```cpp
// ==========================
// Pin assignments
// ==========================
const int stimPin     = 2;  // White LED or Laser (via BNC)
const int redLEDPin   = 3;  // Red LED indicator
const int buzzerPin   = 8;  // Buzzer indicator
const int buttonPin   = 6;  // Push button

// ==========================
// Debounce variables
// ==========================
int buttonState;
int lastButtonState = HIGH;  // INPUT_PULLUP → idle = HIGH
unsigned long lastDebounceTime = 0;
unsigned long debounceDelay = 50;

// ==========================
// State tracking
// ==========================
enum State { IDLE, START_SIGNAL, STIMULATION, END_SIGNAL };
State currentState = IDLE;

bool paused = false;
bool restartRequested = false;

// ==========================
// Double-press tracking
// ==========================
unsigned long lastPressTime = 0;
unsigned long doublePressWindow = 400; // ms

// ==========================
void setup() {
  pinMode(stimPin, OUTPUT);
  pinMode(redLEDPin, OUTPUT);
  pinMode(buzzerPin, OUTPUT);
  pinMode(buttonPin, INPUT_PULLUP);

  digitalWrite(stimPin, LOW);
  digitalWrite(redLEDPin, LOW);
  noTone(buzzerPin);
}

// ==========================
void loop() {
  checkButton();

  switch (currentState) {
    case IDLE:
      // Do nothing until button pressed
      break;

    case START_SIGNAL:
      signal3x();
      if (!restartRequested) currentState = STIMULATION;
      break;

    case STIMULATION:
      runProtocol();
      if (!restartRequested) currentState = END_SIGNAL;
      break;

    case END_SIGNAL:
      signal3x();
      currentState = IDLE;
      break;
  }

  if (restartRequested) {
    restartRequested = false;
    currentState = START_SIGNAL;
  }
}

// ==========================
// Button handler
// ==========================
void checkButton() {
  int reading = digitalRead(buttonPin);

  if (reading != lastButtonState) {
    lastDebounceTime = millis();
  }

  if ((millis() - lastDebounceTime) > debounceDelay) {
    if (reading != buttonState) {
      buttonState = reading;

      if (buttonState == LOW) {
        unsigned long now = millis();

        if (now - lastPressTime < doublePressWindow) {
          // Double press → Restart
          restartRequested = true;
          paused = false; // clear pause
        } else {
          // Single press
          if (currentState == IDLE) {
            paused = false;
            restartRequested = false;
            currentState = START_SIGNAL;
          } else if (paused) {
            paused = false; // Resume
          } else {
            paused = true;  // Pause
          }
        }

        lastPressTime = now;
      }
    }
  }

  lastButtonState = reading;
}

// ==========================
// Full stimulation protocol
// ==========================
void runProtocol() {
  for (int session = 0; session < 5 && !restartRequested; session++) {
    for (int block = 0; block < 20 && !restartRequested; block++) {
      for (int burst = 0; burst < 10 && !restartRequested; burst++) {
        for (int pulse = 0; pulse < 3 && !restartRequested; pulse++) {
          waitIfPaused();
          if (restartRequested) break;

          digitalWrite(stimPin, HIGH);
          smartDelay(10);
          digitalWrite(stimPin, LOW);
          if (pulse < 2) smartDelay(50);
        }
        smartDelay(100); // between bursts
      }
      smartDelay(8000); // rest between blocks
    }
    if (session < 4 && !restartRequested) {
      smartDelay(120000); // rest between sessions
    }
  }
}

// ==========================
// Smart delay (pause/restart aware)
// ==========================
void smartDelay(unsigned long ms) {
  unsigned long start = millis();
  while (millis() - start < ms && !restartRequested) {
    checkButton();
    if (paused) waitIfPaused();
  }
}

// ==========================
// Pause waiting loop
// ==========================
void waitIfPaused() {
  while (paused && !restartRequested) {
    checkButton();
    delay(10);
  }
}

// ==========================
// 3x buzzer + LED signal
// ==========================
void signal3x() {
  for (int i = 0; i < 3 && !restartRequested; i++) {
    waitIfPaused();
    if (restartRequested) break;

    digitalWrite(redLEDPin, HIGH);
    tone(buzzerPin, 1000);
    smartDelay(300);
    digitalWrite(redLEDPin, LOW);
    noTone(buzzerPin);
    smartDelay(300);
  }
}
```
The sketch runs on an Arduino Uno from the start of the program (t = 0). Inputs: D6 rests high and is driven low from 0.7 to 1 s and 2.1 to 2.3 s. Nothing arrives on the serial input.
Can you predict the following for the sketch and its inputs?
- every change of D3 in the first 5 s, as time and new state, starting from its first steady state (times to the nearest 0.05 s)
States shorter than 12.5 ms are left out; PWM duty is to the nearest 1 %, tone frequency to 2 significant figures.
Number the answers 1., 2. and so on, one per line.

1. 0 s low; 0.75 s high; 1.05 s low; 1.35 s high; 1.65 s low; 1.95 s high
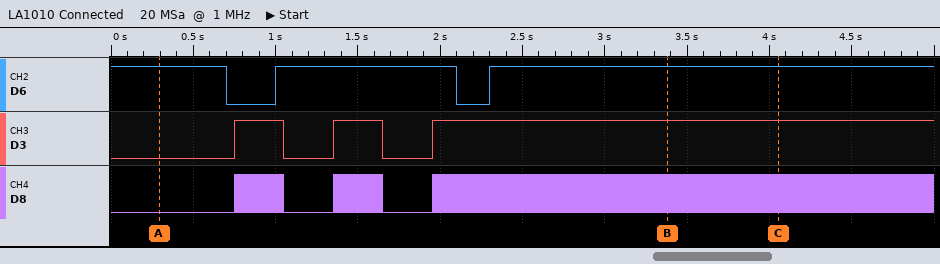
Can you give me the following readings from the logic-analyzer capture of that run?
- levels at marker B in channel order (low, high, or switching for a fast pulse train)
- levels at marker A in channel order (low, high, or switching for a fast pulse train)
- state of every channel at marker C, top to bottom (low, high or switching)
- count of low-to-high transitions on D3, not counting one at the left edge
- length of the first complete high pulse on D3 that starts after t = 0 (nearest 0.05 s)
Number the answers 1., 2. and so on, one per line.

1. D6 high, D3 high, D8 switching
2. D6 high, D3 low, D8 low
3. D6 high, D3 high, D8 switching
4. 3
5. 0.30 s
